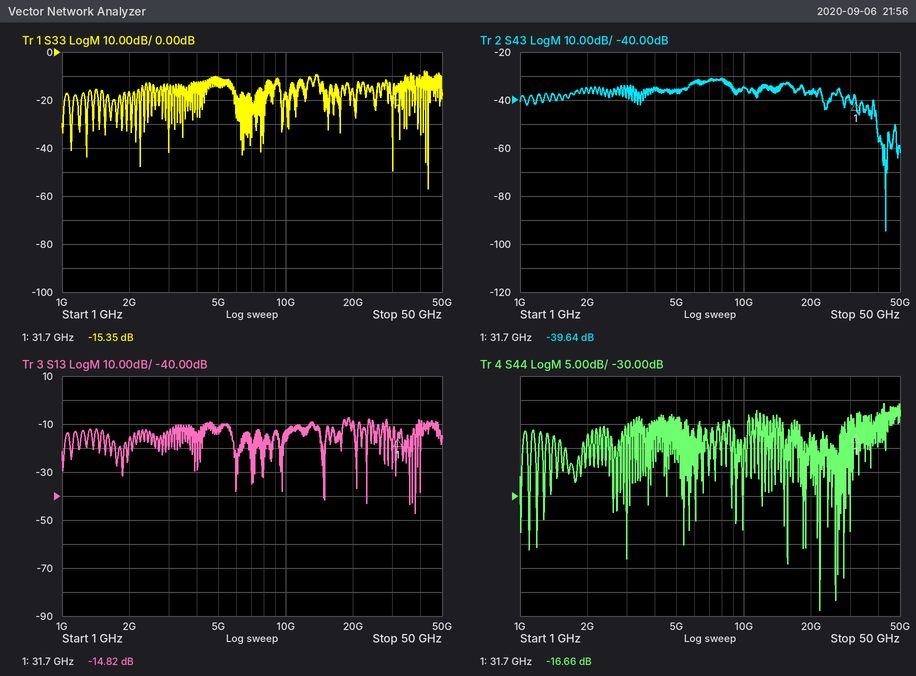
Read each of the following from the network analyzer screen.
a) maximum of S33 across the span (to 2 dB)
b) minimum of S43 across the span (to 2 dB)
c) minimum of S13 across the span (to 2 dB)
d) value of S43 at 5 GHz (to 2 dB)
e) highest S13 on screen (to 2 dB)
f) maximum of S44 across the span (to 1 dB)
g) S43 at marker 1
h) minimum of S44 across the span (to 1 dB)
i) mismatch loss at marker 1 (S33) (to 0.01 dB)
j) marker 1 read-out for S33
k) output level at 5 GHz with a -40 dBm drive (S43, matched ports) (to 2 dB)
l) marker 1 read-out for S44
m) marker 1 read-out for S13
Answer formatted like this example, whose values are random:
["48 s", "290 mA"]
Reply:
["-8 dB", "-94 dB", "-48 dB", "-36 dB", "-8 dB", "-11 dB", "-39.64 dB", "-54 dB", "0.13 dB", "-15.35 dB", "-76 dBm", "-16.66 dB", "-14.82 dB"]
